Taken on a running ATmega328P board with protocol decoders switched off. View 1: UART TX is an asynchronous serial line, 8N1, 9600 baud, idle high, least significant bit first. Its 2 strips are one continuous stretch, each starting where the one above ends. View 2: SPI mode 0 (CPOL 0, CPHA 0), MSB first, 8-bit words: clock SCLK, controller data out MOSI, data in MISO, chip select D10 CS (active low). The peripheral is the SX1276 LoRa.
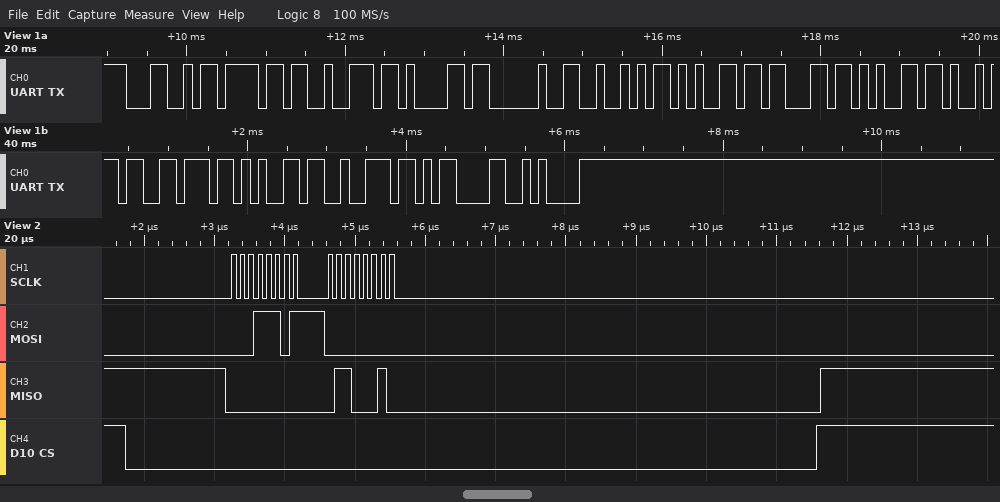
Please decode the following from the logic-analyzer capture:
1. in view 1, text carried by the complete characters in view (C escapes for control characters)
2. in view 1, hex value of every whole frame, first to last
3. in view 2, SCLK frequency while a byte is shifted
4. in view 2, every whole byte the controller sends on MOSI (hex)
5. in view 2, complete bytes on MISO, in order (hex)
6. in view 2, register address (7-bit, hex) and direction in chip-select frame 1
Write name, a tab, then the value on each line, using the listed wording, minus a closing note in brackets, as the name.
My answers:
in view 1, text carried by the complete characters in view	"Lora Receiver\r\n"
in view 1, hex value of every whole frame, first to last	0x4C 0x6F 0x72 0x61 0x20 0x52 0x65 0x63 0x65 0x69 0x76 0x65 0x72 0x0D 0x0A
in view 2, SCLK frequency while a byte is shifted	8 MHz
in view 2, every whole byte the controller sends on MOSI	1D 00
in view 2, complete bytes on MISO, in order	00 62
in view 2, register address (7-bit, hex) and direction in chip-select frame 1	0x1D read
